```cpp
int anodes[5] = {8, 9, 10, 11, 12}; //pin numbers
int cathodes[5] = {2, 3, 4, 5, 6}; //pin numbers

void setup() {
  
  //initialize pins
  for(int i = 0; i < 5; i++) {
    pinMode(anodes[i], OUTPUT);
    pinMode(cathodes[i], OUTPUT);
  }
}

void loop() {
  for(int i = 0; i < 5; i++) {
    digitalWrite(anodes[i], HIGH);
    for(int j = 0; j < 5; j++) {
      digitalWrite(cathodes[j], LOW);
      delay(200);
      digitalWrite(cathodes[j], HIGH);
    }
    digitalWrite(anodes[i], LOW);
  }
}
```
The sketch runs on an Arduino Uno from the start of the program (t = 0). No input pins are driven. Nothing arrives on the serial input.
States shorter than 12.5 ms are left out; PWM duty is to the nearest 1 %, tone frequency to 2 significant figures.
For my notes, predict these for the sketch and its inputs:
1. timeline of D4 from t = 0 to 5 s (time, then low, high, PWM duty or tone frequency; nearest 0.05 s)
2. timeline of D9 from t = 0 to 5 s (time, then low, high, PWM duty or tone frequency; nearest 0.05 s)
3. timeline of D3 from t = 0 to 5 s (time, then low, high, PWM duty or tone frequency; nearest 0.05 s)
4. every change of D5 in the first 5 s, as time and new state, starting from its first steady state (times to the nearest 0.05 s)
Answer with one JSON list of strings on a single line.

["0 s low; 0.6 s high; 1.4 s low; 1.6 s high; 2.4 s low; 2.6 s high; 3.4 s low; 3.6 s high; 4.4 s low; 4.6 s high", "0 s low; 1 s high; 2 s low", "0 s low; 0.4 s high; 1.2 s low; 1.4 s high; 2.2 s low; 2.4 s high; 3.2 s low; 3.4 s high; 4.2 s low; 4.4 s high", "0 s low; 0.8 s high; 1.6 s low; 1.8 s high; 2.6 s low; 2.8 s high; 3.6 s low; 3.8 s high; 4.6 s low; 4.8 s high"]
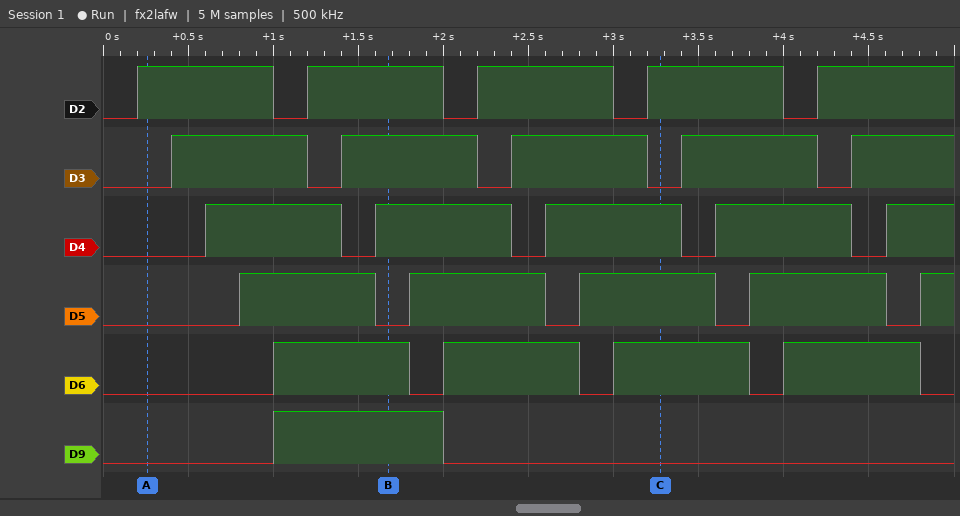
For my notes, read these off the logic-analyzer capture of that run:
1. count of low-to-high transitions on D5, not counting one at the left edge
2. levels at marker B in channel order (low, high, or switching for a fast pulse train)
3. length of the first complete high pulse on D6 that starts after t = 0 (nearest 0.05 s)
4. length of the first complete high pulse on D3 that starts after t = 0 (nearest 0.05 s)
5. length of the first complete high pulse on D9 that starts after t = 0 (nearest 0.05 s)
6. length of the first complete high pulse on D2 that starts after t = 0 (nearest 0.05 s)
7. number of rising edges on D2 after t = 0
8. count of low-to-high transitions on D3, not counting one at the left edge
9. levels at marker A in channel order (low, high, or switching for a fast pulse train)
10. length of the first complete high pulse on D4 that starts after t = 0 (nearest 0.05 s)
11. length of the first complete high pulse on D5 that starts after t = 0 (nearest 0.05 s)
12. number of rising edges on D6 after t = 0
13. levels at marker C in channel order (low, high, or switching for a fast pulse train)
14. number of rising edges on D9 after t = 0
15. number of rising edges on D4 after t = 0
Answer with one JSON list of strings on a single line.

["5", "D2 high, D3 high, D4 high, D5 low, D6 high, D9 high", "0.80 s", "0.80 s", "1.00 s", "0.80 s", "5", "5", "D2 high, D3 low, D4 low, D5 low, D6 low, D9 low", "0.80 s", "0.80 s", "4", "D2 high, D3 low, D4 high, D5 high, D6 high, D9 low", "1", "5"]
